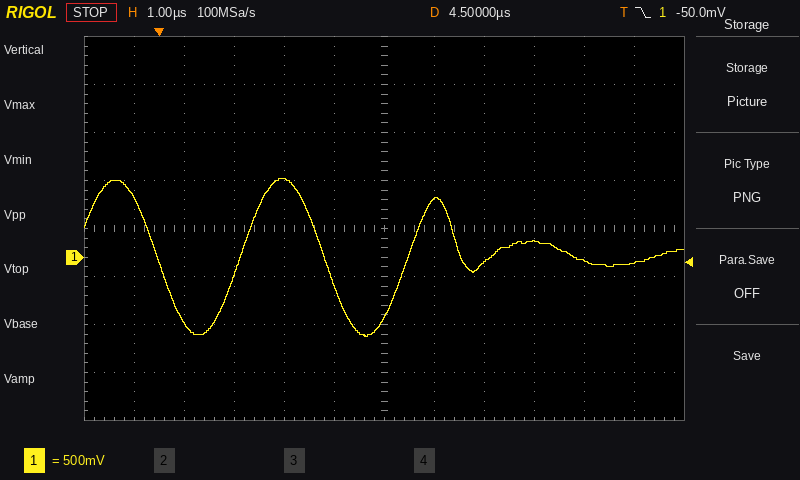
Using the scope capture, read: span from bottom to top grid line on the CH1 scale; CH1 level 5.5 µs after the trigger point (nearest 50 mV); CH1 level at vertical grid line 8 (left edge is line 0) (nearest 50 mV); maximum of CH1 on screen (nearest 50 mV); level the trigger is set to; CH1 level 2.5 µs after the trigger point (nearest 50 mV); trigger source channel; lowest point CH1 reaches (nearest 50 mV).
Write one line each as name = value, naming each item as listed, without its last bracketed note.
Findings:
span from bottom to top grid line on the CH1 scale = 4 V
CH1 level 5.5 µs after the trigger point = 600 mV
CH1 level at vertical grid line 8 (left edge is line 0) = -50 mV
maximum of CH1 on screen = 800 mV
level the trigger is set to = -50.0 mV
CH1 level 2.5 µs after the trigger point = 800 mV
trigger source channel = CH1
lowest point CH1 reaches = -800 mV
